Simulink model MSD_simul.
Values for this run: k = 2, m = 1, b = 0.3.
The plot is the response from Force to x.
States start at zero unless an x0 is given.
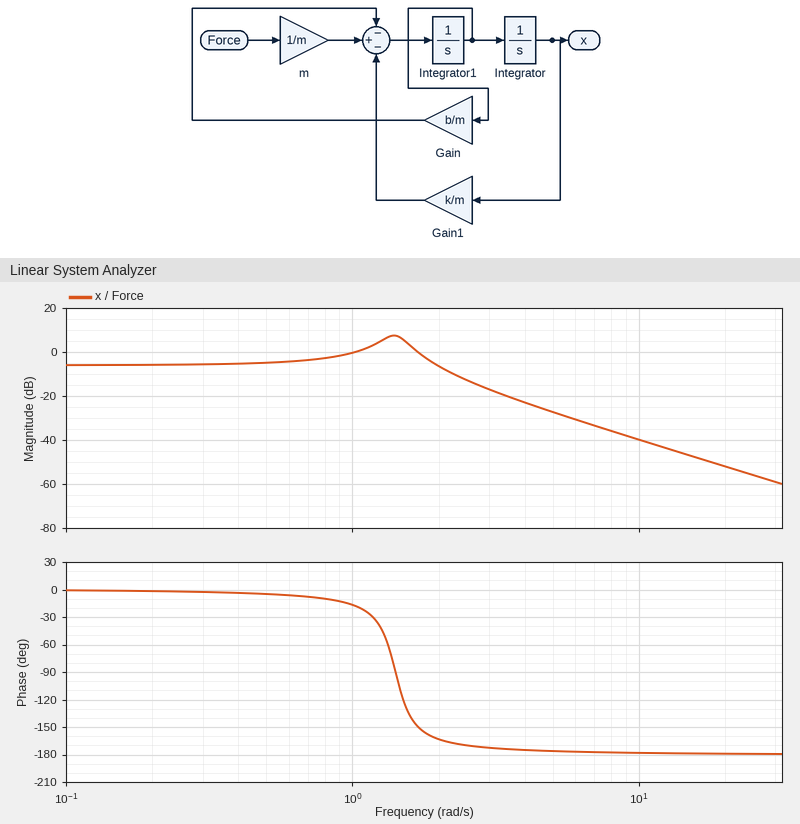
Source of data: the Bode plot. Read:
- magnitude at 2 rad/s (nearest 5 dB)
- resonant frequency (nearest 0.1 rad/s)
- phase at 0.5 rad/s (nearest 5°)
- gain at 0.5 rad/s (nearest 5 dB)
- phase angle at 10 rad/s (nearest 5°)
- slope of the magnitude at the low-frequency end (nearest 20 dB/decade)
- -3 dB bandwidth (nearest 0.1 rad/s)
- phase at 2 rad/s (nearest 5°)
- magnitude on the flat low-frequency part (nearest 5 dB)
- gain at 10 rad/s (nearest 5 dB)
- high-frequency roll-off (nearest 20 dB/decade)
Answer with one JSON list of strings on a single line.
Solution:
["-5 dB", "1.4 rad/s", "-5°", "-5 dB", "-180°", "0 dB/decade", "2.2 rad/s", "-165°", "-5 dB", "-40 dB", "-40 dB/decade"]
